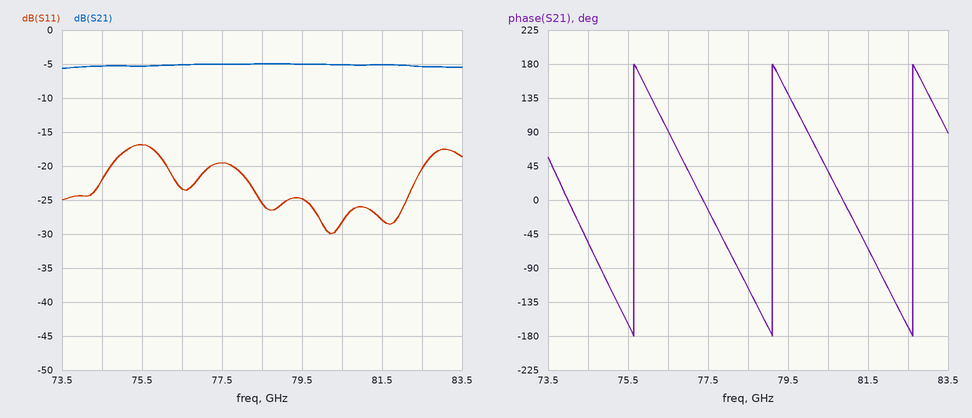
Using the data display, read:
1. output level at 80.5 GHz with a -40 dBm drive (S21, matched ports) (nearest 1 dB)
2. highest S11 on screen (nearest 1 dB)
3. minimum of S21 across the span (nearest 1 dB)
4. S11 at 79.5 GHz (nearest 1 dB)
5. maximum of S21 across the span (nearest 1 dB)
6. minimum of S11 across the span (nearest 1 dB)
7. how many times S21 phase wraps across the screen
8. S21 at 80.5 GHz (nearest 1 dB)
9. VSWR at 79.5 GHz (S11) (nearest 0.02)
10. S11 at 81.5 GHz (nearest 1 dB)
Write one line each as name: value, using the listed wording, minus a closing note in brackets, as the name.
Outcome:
output level at 80.5 GHz with a -40 dBm drive (S21, matched ports): -45 dBm
highest S11 on screen: -17 dB
minimum of S21 across the span: -6 dB
S11 at 79.5 GHz: -25 dB
maximum of S21 across the span: -5 dB
minimum of S11 across the span: -30 dB
how many times S21 phase wraps across the screen: 3
S21 at 80.5 GHz: -5 dB
VSWR at 79.5 GHz (S11): 1.12
S11 at 81.5 GHz: -28 dB
